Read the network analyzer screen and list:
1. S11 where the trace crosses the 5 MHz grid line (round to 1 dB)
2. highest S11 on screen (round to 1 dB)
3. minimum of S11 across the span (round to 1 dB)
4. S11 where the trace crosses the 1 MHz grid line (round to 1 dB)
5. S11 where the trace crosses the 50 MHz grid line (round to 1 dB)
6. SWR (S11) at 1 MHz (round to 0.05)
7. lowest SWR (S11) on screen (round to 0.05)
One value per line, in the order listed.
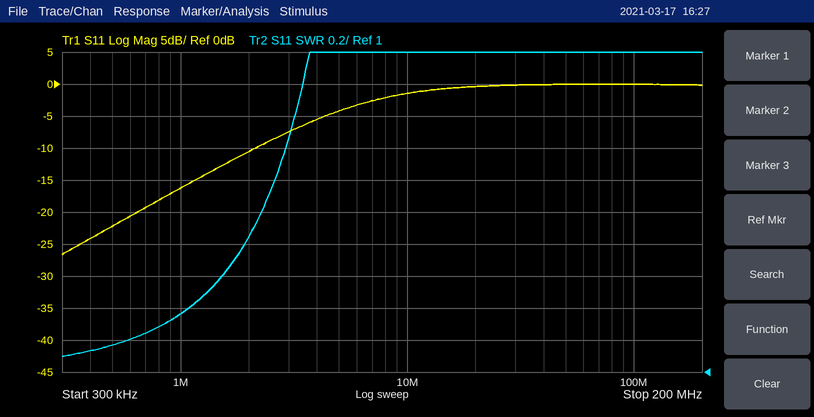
-4 dB
0 dB
-27 dB
-16 dB
0 dB
1.35
1.10
